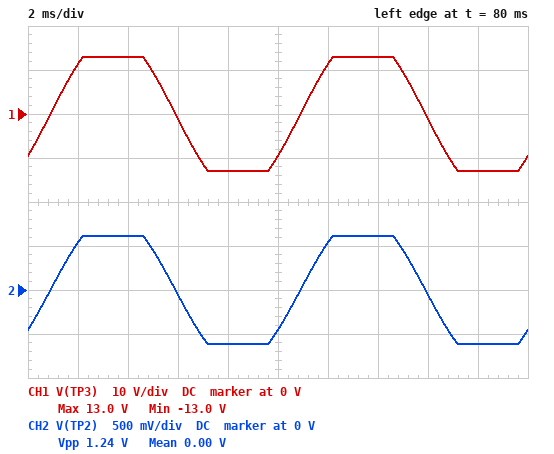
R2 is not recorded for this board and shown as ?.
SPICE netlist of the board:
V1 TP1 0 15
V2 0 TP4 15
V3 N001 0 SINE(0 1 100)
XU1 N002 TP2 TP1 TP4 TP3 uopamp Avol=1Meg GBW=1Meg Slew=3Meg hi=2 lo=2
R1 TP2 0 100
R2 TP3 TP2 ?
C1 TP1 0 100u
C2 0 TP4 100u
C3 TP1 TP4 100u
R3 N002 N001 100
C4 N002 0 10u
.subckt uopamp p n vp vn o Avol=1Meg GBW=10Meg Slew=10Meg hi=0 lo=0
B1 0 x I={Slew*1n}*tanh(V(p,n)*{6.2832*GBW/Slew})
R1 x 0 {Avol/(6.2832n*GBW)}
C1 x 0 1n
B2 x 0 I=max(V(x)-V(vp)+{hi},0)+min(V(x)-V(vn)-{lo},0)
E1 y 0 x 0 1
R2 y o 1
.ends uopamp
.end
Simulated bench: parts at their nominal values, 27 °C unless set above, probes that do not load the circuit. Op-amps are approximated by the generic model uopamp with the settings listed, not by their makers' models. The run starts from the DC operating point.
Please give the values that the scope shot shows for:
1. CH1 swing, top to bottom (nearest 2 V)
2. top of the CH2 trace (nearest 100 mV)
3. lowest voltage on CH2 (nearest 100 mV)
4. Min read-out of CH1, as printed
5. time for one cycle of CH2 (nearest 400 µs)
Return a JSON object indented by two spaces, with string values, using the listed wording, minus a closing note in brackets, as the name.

{
  "CH1 swing, top to bottom": "26 V",
  "top of the CH2 trace": "600 mV",
  "lowest voltage on CH2": "-600 mV",
  "Min read-out of CH1, as printed": "-13.0 V",
  "time for one cycle of CH2": "10.0 ms"
}
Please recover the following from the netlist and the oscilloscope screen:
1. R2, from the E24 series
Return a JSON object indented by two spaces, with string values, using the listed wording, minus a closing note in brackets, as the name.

{
  "R2, from the E24 series": "2 kΩ"
}
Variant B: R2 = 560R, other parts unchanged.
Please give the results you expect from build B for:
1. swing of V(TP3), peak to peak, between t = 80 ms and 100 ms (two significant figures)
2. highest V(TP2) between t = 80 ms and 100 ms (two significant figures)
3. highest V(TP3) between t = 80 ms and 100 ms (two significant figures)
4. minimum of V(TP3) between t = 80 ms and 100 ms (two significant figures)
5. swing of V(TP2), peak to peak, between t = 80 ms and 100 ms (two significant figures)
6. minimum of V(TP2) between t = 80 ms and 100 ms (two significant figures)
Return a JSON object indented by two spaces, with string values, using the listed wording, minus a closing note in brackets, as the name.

{
  "swing of V(TP3), peak to peak, between t = 80 ms and 100 ms": "11 V",
  "highest V(TP2) between t = 80 ms and 100 ms": "850 mV",
  "highest V(TP3) between t = 80 ms and 100 ms": "5.6 V",
  "minimum of V(TP3) between t = 80 ms and 100 ms": "-5.6 V",
  "swing of V(TP2), peak to peak, between t = 80 ms and 100 ms": "1.7 V",
  "minimum of V(TP2) between t = 80 ms and 100 ms": "-850 mV"
}
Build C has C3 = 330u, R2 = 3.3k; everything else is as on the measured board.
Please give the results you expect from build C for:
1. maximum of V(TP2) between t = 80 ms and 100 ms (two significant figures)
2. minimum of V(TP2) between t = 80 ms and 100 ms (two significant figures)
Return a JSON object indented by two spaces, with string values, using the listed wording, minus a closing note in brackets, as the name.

{
  "maximum of V(TP2) between t = 80 ms and 100 ms": "380 mV",
  "minimum of V(TP2) between t = 80 ms and 100 ms": "-380 mV"
}
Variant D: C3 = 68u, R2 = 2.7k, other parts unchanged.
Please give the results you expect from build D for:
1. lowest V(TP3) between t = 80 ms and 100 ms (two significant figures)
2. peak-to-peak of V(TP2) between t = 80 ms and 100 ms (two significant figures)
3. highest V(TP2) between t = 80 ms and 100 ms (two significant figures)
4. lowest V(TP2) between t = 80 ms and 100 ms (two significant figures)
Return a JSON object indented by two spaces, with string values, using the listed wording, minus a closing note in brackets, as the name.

{
  "lowest V(TP3) between t = 80 ms and 100 ms": "-13 V",
  "peak-to-peak of V(TP2) between t = 80 ms and 100 ms": "930 mV",
  "highest V(TP2) between t = 80 ms and 100 ms": "460 mV",
  "lowest V(TP2) between t = 80 ms and 100 ms": "-460 mV"
}
